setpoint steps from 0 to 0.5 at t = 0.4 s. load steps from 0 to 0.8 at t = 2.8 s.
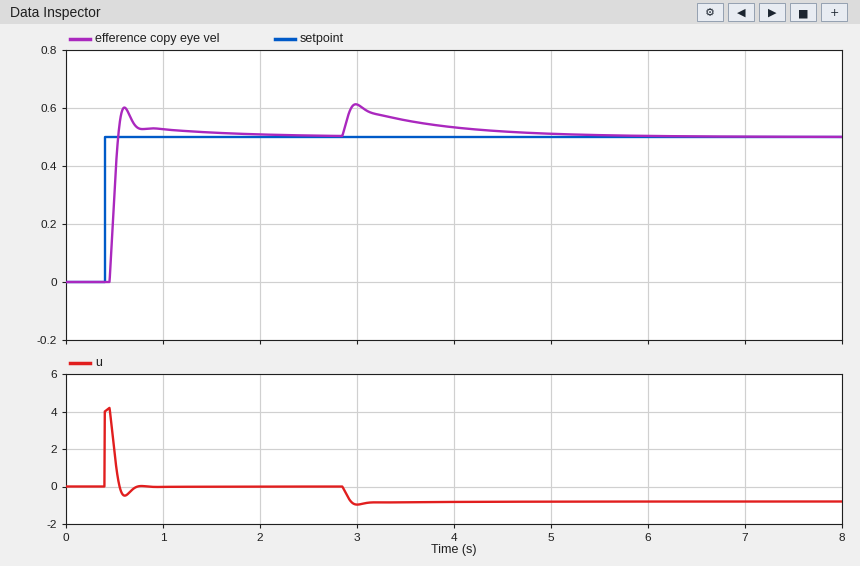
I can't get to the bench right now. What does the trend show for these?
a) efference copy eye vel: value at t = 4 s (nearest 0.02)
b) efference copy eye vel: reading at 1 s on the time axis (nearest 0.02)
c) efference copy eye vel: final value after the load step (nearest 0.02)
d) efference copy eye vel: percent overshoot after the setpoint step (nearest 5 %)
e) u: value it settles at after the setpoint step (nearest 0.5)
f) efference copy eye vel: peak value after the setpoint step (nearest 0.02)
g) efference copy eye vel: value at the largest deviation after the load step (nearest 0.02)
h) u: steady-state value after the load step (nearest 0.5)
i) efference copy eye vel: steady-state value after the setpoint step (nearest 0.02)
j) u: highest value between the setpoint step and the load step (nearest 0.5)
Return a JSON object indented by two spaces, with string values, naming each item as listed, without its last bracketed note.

{
  "efference copy eye vel: value at t = 4 s": "0.54",
  "efference copy eye vel: reading at 1 s on the time axis": "0.52",
  "efference copy eye vel: final value after the load step": "0.50",
  "efference copy eye vel: percent overshoot after the setpoint step": "20 %",
  "u: value it settles at after the setpoint step": "0.0",
  "efference copy eye vel: peak value after the setpoint step": "0.60",
  "efference copy eye vel: value at the largest deviation after the load step": "0.62",
  "u: steady-state value after the load step": "-1.0",
  "efference copy eye vel: steady-state value after the setpoint step": "0.50",
  "u: highest value between the setpoint step and the load step": "4.0"
}
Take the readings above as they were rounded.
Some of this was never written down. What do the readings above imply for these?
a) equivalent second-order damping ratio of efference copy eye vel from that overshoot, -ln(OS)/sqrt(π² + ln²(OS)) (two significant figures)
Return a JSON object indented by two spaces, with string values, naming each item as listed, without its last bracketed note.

{
  "equivalent second-order damping ratio of efference copy eye vel from that overshoot, -ln(OS)/sqrt(π² + ln²(OS))": "0.46"
}
